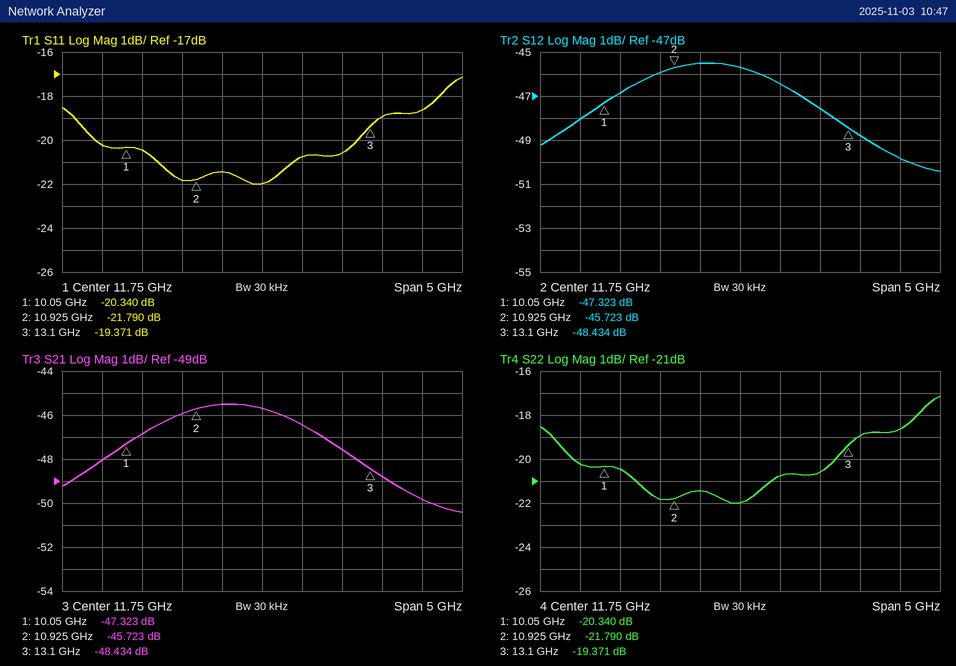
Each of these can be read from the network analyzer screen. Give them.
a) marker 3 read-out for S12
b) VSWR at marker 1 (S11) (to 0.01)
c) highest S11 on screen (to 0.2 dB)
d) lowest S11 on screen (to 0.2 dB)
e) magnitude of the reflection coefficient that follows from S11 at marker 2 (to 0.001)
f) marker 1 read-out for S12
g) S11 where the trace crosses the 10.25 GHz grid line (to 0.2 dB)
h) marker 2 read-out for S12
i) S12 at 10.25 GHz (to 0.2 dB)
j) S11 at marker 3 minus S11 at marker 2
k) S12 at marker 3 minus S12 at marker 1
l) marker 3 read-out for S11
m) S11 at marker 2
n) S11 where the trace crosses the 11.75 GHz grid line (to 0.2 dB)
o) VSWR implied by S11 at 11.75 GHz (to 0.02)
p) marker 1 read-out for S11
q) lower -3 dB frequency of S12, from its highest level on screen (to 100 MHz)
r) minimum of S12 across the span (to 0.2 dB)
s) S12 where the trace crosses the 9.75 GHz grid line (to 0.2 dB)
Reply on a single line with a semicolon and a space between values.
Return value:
-48.434 dB; 1.21; -17.2 dB; -22.0 dB; 0.081; -47.323 dB; -20.4 dB; -45.723 dB; -46.8 dB; 2.419 dB; -1.111 dB; -19.371 dB; -21.790 dB; -22.0 dB; 1.18; -20.340 dB; 9.6 GHz; -50.4 dB; -48.0 dB
